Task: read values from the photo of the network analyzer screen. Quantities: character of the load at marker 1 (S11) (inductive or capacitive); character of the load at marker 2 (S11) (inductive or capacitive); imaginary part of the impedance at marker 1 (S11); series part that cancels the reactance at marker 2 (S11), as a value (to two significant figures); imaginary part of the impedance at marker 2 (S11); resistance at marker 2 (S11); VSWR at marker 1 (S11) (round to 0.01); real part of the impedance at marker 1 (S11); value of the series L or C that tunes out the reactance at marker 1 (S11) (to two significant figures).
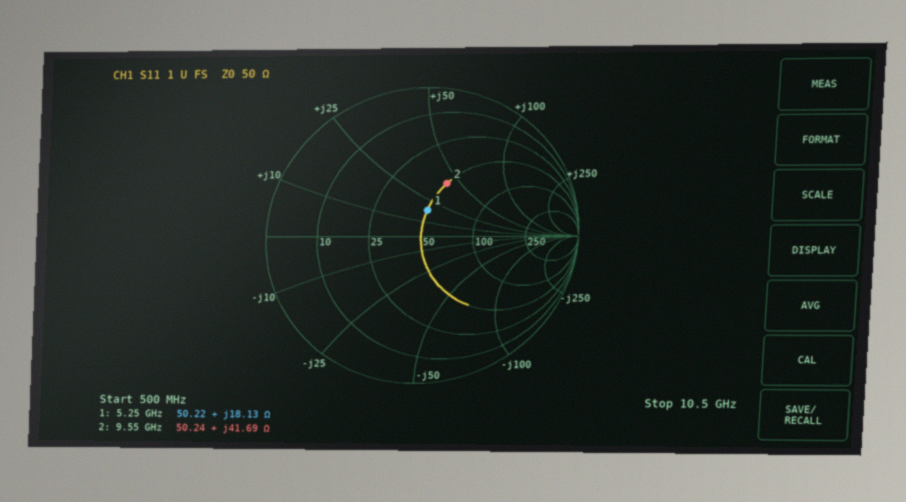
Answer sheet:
inductive
inductive
+18.13 Ω
400 fF
+41.69 Ω
50.24 Ω
1.43
50.22 Ω
1.7 pF
